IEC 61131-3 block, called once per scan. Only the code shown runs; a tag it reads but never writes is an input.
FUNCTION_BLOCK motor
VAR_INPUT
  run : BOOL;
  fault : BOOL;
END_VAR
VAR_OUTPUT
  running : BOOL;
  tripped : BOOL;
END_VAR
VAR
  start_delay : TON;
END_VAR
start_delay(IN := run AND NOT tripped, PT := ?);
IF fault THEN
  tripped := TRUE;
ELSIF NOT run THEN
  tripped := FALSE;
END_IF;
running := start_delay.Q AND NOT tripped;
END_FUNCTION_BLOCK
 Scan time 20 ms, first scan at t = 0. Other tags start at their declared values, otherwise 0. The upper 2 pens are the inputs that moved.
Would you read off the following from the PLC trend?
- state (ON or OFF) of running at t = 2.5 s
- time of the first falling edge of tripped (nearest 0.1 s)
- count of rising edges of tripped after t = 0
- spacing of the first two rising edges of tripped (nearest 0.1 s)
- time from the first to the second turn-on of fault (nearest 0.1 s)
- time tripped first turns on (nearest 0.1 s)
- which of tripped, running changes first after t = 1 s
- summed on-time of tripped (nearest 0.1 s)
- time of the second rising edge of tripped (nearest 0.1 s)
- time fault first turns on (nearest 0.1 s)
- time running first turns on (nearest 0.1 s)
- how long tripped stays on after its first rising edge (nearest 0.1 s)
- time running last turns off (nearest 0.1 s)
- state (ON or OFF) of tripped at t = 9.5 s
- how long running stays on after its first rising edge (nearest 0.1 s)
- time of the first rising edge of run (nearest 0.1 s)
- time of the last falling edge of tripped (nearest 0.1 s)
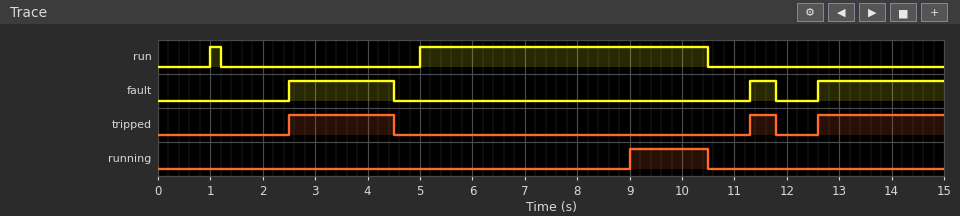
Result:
OFF
4.5 s
3
8.8 s
8.8 s
2.5 s
tripped
4.9 s
11.3 s
2.5 s
9.0 s
2.0 s
10.5 s
OFF
1.5 s
1.0 s
11.8 s
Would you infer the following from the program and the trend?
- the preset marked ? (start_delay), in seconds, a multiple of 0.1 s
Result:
4.0 s
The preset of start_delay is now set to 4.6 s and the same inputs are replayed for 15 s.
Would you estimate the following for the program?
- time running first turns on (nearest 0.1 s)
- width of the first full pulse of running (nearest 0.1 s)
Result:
9.6 s
0.9 s
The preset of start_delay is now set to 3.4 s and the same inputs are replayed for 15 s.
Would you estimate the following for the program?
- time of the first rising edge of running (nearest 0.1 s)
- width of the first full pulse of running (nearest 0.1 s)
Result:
8.4 s
2.1 s
